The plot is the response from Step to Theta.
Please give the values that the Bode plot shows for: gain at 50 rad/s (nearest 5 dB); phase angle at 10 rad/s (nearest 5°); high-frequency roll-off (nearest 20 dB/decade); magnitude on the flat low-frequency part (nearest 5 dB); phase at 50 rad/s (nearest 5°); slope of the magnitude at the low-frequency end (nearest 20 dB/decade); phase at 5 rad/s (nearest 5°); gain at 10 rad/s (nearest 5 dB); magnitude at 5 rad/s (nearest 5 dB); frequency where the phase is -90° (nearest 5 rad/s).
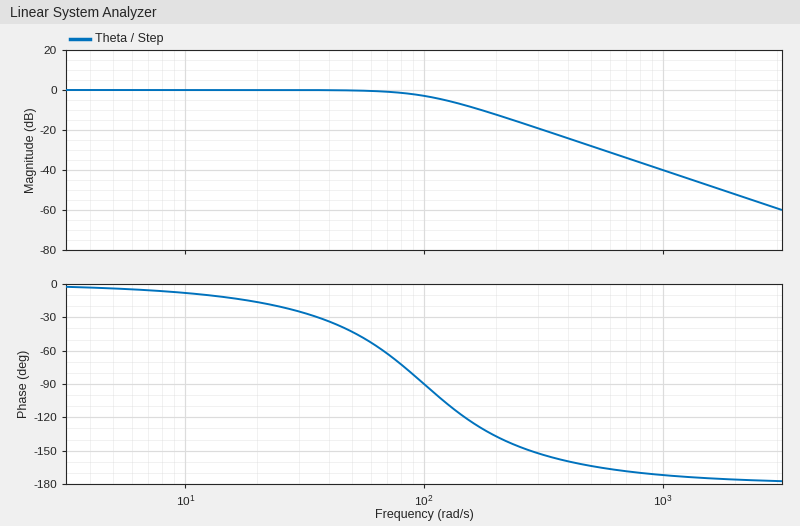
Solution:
0 dB
-10°
-40 dB/decade
0 dB
-45°
0 dB/decade
-5°
0 dB
0 dB
100 rad/s
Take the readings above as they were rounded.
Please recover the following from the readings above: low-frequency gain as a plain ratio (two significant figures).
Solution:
1.0
